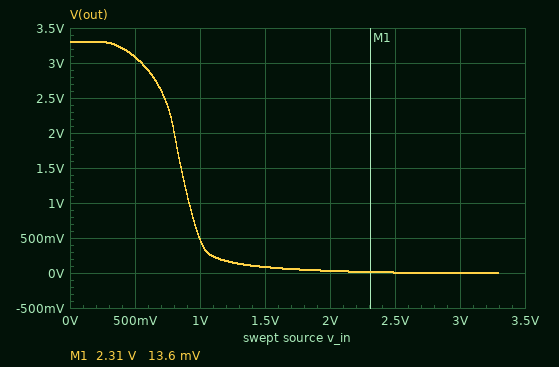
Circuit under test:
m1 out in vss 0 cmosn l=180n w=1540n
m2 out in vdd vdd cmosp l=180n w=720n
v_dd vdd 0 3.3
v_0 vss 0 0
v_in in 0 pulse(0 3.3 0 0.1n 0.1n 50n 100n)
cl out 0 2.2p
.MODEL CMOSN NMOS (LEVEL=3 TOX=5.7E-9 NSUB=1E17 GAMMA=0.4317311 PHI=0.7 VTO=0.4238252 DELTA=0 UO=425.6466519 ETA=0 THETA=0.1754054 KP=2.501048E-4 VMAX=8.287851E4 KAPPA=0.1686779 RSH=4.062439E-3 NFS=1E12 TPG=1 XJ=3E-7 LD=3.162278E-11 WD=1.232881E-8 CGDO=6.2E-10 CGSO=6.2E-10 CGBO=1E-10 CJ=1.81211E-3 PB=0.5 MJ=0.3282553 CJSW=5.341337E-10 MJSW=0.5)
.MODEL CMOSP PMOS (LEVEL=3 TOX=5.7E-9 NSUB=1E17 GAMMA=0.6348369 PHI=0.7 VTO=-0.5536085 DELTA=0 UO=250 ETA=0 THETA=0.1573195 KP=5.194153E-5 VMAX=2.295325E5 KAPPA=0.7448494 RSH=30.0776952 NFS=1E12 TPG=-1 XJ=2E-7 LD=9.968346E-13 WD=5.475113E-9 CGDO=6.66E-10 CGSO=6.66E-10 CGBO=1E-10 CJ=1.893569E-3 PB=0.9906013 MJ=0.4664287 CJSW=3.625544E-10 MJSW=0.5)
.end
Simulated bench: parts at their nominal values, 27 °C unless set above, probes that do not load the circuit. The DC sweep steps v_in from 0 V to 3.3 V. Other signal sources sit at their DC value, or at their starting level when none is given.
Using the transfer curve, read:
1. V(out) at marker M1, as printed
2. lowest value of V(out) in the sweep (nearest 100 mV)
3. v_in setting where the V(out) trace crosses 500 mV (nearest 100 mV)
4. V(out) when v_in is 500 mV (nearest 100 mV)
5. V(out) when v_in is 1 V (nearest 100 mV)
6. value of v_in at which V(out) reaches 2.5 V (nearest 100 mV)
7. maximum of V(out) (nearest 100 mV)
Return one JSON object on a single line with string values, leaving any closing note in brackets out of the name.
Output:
{"V(out) at marker M1, as printed": "13.6 mV", "lowest value of V(out) in the sweep": "0 V", "v_in setting where the V(out) trace crosses 500 mV": "1.0 V", "V(out) when v_in is 500 mV": "3.1 V", "V(out) when v_in is 1 V": "500 mV", "value of v_in at which V(out) reaches 2.5 V": "700 mV", "maximum of V(out)": "3.3 V"}
